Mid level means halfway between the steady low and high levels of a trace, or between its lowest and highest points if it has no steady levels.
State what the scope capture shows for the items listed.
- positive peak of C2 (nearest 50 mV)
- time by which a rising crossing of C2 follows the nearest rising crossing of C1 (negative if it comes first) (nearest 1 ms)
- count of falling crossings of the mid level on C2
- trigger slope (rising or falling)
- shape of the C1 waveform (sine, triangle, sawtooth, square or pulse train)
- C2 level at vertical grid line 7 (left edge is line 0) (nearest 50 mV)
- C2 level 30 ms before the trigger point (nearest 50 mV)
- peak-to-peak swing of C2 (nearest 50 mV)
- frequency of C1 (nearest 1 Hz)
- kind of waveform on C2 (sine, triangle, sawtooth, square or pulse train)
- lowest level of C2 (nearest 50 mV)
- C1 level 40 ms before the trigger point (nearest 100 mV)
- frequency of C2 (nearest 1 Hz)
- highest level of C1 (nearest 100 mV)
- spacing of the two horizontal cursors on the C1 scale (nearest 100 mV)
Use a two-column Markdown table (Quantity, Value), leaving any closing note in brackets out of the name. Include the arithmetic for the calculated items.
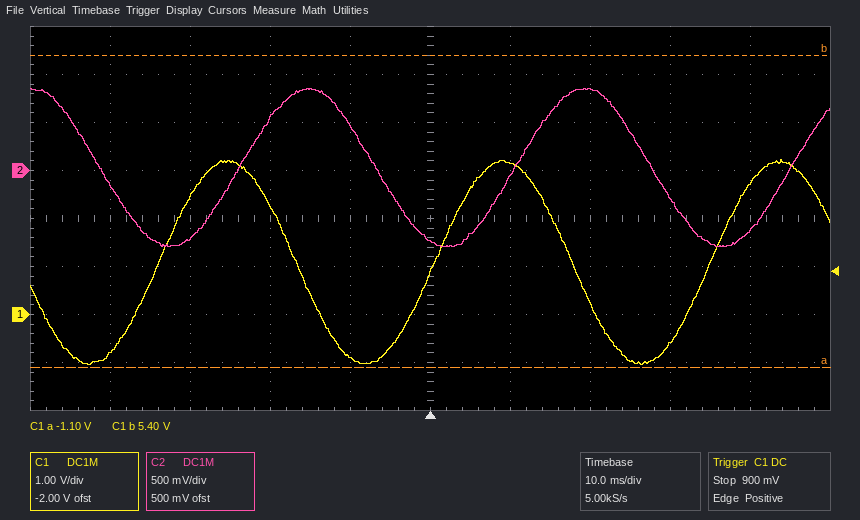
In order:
| Quantity | Value |
|---|---|
| positive peak of C2 | 850 mV |
| time by which a rising crossing of C2 follows the nearest rising crossing of C1 (negative if it comes first) | +10 ms |
| count of falling crossings of the mid level on C2 | 3 |
| trigger slope | rising |
| shape of the C1 waveform | sine |
| C2 level at vertical grid line 7 (left edge is line 0) | 850 mV |
| C2 level 30 ms before the trigger point | -700 mV |
| peak-to-peak swing of C2 | 850 mV − (-800 mV) = 1.65 V |
| frequency of C1 | 29 Hz |
| kind of waveform on C2 | sine |
| lowest level of C2 | -800 mV |
| C1 level 40 ms before the trigger point | -800 mV |
| frequency of C2 | 29 Hz |
| highest level of C1 | 3.2 V |
| spacing of the two horizontal cursors on the C1 scale | 6.5 V |
